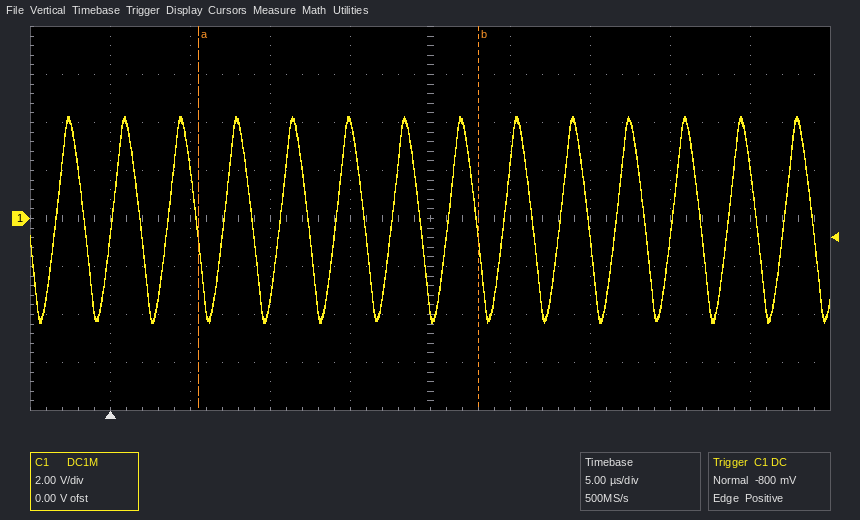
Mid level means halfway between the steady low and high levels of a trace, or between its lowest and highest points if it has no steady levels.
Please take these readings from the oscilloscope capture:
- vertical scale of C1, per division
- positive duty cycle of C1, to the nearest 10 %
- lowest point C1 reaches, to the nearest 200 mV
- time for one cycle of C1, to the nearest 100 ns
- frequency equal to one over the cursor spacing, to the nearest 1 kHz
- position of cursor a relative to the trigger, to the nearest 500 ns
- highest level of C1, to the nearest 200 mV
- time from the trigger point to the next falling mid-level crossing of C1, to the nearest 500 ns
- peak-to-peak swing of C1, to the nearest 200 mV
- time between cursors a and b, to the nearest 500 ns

2 V
50 %
-4.4 V
3.5 µs
57 kHz
+5.5 µs
4.2 V
2.0 µs
8.6 V
17.5 µs
